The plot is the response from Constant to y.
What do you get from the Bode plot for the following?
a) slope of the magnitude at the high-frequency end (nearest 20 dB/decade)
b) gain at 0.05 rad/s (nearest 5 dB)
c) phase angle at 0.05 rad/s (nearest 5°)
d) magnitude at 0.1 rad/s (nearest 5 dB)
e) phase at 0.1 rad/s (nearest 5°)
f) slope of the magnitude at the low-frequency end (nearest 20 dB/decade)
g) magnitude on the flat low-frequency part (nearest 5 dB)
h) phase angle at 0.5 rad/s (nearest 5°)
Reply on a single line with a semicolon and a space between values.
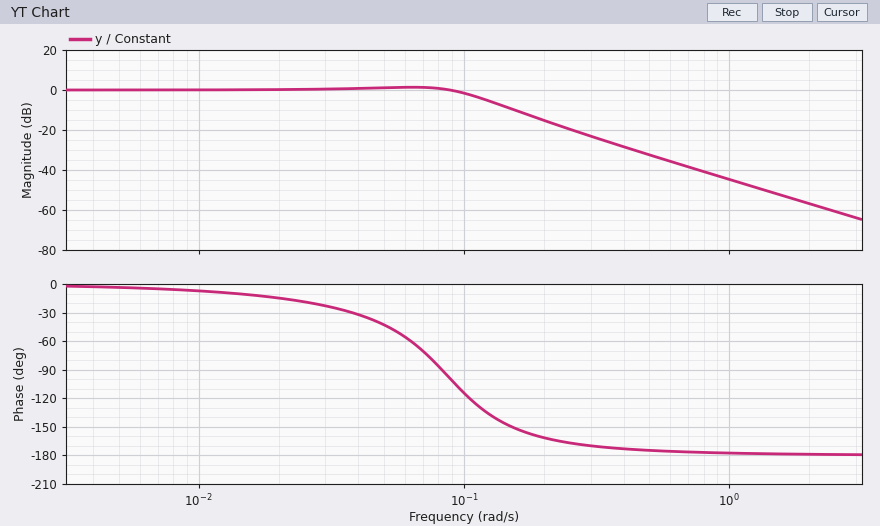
-40 dB/decade; 0 dB; -45°; 0 dB; -115°; 0 dB/decade; 0 dB; -175°
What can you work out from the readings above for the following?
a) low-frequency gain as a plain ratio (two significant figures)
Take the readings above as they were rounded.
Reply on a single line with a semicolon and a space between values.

1.0
